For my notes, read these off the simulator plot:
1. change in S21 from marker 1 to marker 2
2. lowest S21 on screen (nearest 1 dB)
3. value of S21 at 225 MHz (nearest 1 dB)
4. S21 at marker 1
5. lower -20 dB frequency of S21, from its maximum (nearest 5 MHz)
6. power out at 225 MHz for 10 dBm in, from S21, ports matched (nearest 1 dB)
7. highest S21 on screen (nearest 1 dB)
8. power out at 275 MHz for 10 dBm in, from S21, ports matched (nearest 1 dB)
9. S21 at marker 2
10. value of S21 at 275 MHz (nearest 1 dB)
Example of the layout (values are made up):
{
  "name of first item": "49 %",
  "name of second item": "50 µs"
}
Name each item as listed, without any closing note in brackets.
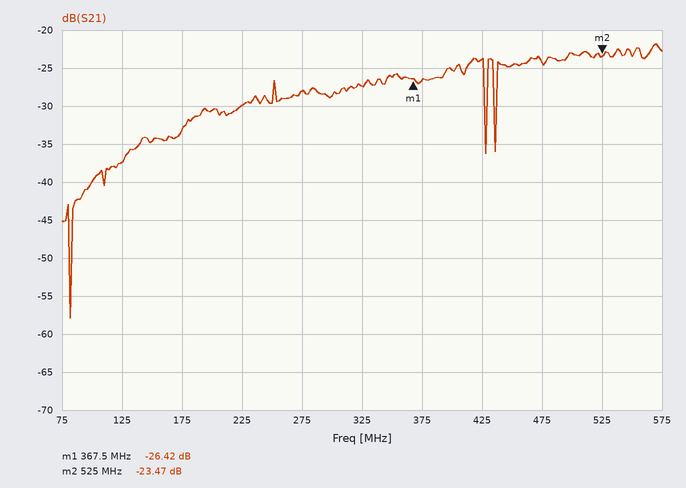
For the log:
{
  "change in S21 from marker 1 to marker 2": "2.95 dB",
  "lowest S21 on screen": "-58 dB",
  "value of S21 at 225 MHz": "-30 dB",
  "S21 at marker 1": "-26.42 dB",
  "lower -20 dB frequency of S21, from its maximum": "90 MHz",
  "power out at 225 MHz for 10 dBm in, from S21, ports matched": "-20 dBm",
  "highest S21 on screen": "-22 dB",
  "power out at 275 MHz for 10 dBm in, from S21, ports matched": "-18 dBm",
  "S21 at marker 2": "-23.47 dB",
  "value of S21 at 275 MHz": "-28 dB"
}
